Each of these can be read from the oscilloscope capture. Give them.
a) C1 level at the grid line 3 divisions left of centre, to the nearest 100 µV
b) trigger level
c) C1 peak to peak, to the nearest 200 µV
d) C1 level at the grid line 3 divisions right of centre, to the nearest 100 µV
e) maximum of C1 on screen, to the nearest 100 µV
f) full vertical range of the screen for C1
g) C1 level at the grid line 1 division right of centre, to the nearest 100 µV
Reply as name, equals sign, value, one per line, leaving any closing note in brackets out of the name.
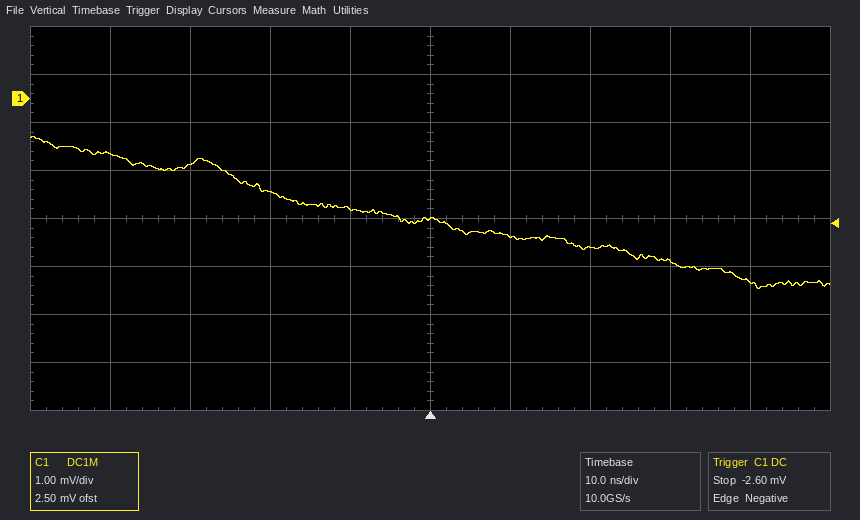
C1 level at the grid line 3 divisions left of centre, to the nearest 100 µV = -1.4 mV
trigger level = -2.60 mV
C1 peak to peak, to the nearest 200 µV = 3.2 mV
C1 level at the grid line 3 divisions right of centre, to the nearest 100 µV = -3.4 mV
maximum of C1 on screen, to the nearest 100 µV = -800 µV
full vertical range of the screen for C1 = 8 mV
C1 level at the grid line 1 division right of centre, to the nearest 100 µV = -2.9 mV
